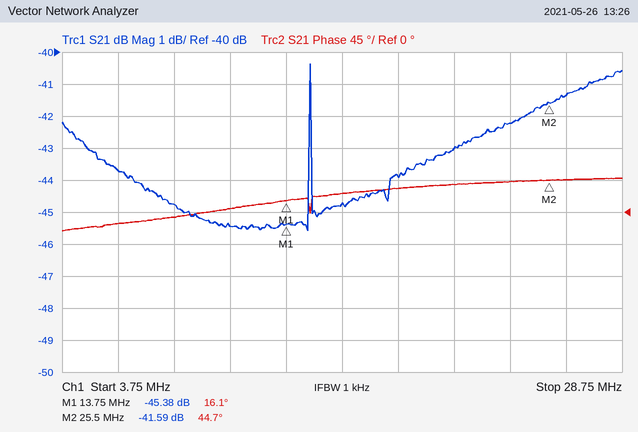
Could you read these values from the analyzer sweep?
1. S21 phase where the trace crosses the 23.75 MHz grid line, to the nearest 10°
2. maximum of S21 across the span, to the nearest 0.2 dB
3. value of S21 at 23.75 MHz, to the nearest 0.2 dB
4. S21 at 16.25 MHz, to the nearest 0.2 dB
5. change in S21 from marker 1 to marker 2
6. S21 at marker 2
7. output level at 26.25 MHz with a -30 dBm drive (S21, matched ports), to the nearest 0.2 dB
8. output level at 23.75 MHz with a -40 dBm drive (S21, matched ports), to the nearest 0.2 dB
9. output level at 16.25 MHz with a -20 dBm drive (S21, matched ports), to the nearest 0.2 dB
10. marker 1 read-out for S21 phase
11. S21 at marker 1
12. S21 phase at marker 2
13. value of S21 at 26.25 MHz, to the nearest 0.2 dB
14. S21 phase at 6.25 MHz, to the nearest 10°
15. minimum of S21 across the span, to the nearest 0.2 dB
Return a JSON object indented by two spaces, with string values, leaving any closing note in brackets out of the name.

{
  "S21 phase where the trace crosses the 23.75 MHz grid line, to the nearest 10°": "40°",
  "maximum of S21 across the span, to the nearest 0.2 dB": "-40.4 dB",
  "value of S21 at 23.75 MHz, to the nearest 0.2 dB": "-42.2 dB",
  "S21 at 16.25 MHz, to the nearest 0.2 dB": "-44.8 dB",
  "change in S21 from marker 1 to marker 2": "3.79 dB",
  "S21 at marker 2": "-41.59 dB",
  "output level at 26.25 MHz with a -30 dBm drive (S21, matched ports), to the nearest 0.2 dB": "-71.4 dBm",
  "output level at 23.75 MHz with a -40 dBm drive (S21, matched ports), to the nearest 0.2 dB": "-82.2 dBm",
  "output level at 16.25 MHz with a -20 dBm drive (S21, matched ports), to the nearest 0.2 dB": "-64.8 dBm",
  "marker 1 read-out for S21 phase": "16.1°",
  "S21 at marker 1": "-45.38 dB",
  "S21 phase at marker 2": "44.7°",
  "value of S21 at 26.25 MHz, to the nearest 0.2 dB": "-41.4 dB",
  "S21 phase at 6.25 MHz, to the nearest 10°": "-20°",
  "minimum of S21 across the span, to the nearest 0.2 dB": "-45.6 dB"
}
